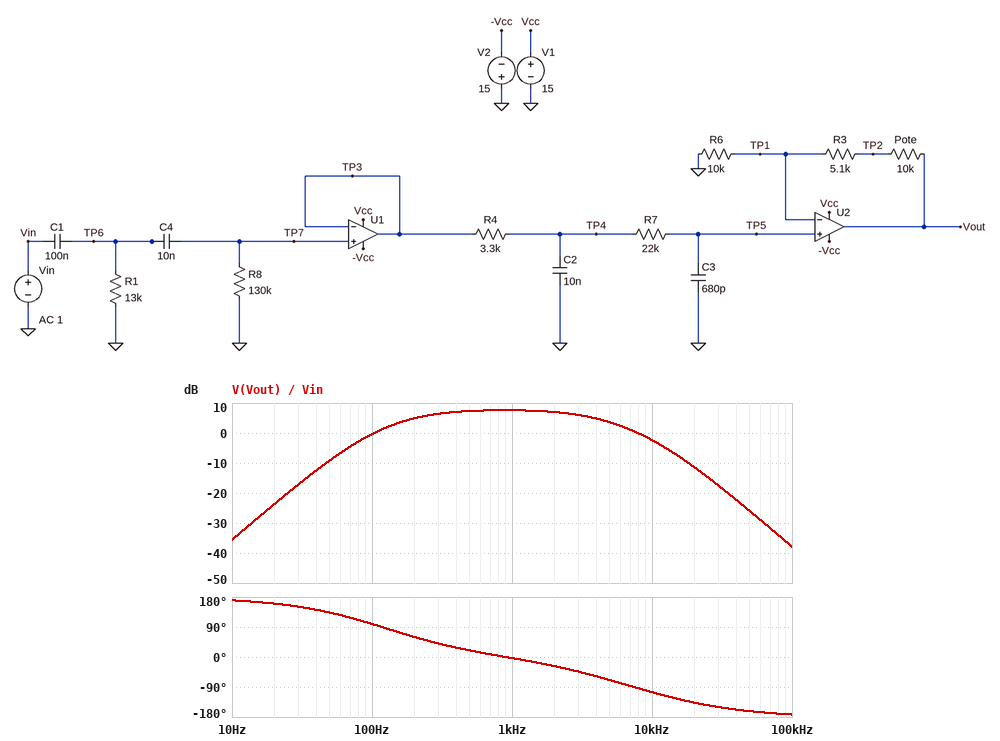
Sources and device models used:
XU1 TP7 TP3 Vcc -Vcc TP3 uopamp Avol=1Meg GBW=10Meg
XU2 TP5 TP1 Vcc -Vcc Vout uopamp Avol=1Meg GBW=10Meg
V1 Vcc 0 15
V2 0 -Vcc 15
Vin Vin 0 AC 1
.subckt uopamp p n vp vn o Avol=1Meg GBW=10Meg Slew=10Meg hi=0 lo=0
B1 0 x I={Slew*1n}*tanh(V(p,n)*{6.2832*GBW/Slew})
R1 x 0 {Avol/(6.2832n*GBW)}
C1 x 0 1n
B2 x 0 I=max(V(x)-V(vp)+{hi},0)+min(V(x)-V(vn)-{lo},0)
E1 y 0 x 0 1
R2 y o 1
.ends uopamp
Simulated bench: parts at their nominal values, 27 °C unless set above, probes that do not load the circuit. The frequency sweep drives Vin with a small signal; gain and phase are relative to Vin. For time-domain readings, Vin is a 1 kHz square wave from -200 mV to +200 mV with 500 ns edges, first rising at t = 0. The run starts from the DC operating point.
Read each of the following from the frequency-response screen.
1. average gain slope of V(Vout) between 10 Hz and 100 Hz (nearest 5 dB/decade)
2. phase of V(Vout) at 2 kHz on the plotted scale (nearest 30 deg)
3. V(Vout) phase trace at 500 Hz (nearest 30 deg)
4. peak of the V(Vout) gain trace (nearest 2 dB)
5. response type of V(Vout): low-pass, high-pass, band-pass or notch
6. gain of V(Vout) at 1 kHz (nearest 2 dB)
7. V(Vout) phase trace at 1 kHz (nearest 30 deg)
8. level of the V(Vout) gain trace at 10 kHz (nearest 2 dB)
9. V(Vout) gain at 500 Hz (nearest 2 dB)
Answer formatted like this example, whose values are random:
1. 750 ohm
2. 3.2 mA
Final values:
1. 35 dB/decade
2. -30 deg
3. 30 deg
4. 8 dB
5. band-pass
6. 8 dB
7. 0 deg
8. -2 dB
9. 8 dB
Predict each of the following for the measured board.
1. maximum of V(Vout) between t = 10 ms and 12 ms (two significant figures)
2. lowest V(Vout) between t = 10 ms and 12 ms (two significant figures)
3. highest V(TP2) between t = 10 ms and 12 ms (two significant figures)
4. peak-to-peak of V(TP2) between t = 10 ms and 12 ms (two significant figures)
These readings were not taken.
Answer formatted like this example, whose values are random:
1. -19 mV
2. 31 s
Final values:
1. 570 mV
2. -570 mV
3. 340 mV
4. 690 mV
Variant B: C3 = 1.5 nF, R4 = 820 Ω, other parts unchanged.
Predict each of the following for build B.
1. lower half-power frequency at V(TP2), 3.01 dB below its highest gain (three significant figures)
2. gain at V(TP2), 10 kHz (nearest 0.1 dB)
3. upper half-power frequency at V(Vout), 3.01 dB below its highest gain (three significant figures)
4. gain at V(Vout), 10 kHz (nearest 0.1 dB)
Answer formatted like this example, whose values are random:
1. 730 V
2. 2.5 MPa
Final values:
1. 190 Hz
2. -4.9 dB
3. 4.73 kHz
4. -0.5 dB
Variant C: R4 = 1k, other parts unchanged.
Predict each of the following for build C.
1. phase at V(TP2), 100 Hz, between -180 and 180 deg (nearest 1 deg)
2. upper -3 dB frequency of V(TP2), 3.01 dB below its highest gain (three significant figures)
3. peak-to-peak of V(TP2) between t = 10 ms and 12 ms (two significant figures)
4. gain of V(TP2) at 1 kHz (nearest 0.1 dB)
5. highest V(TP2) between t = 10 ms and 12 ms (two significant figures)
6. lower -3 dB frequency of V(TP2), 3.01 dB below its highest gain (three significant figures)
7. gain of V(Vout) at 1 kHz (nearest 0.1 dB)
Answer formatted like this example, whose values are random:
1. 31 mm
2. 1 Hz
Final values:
1. 100 deg
2. 8.14 kHz
3. 750 mV
4. 3.4 dB
5. 380 mV
6. 196 Hz
7. 7.8 dB
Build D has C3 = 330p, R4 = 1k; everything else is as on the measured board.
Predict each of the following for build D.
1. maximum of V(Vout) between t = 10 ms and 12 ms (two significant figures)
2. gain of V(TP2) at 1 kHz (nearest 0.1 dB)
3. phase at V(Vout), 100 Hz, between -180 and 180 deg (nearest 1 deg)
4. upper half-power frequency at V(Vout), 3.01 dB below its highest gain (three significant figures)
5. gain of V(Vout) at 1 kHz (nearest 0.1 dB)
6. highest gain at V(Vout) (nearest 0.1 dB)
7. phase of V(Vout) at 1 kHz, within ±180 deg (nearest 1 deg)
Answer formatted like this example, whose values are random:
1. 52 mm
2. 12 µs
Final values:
1. 640 mV
2. 3.4 dB
3. 100 deg
4. 11.8 kHz
5. 7.8 dB
6. 7.9 dB
7. 8 deg
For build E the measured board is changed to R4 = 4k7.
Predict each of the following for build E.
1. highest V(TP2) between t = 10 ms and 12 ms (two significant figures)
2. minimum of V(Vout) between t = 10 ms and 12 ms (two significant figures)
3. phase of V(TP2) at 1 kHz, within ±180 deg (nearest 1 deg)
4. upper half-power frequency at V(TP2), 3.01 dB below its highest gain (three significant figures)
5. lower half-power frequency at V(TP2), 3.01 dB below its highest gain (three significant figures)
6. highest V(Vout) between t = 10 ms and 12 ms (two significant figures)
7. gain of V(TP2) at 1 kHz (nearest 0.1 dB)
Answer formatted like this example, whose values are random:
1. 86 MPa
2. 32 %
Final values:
1. 330 mV
2. -540 mV
3. -8 deg
4. 3.23 kHz
5. 184 Hz
6. 540 mV
7. 3.0 dB
